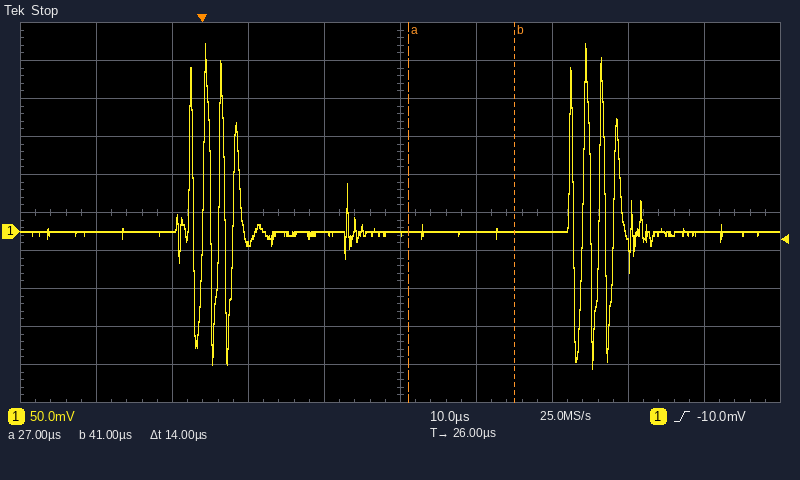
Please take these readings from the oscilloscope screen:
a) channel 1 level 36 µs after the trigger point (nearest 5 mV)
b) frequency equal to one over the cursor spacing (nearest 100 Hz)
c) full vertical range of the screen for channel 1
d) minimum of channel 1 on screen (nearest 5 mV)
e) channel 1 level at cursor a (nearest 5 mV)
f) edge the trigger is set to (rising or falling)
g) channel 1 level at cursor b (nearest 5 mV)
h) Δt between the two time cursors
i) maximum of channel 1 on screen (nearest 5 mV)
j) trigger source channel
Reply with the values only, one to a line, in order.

0 mV
71.4 kHz
500 mV
-180 mV
0 mV
rising
0 mV
14 µs
245 mV
channel 1
